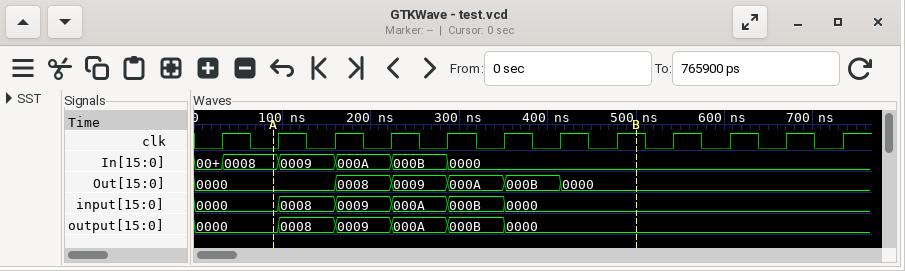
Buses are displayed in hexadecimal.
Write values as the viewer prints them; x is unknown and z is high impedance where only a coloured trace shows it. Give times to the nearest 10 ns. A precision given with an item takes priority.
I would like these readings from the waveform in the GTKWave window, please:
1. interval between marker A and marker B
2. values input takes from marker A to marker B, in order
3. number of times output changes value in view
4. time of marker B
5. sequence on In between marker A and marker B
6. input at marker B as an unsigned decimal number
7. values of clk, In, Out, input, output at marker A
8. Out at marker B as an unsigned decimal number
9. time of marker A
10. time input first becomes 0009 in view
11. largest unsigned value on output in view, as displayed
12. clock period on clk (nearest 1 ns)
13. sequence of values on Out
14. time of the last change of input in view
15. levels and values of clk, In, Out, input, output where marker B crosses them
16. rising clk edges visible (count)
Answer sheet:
410 ns
0000, 0008, 0009, 000A, 000B, 0000
5
500 ns
0008, 0009, 000A, 000B, 0000
0
clk=0, In=0008, Out=0000, input=0000, output=0000
0
90 ns
160 ns
000B
64 ns
0000, 0008, 0009, 000A, 000B, 0000
350 ns
clk=1, In=0000, Out=0000, input=0000, output=0000
12
